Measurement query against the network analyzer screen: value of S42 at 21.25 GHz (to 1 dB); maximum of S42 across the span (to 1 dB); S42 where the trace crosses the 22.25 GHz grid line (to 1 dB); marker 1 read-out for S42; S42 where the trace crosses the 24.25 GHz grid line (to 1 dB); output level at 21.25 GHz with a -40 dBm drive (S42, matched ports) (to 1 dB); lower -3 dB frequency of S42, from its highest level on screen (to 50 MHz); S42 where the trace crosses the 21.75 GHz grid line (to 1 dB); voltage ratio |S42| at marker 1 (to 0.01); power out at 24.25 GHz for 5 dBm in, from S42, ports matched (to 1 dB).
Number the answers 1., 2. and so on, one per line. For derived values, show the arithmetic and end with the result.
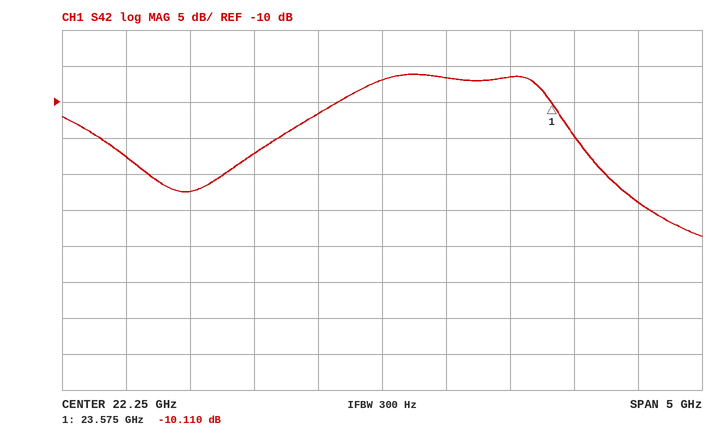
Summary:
1. -17 dB
2. -6 dB
3. -7 dB
4. -10.110 dB
5. -24 dB
6. -40 dBm + (-17 dB) = -57 dBm
7. 22.00 GHz
8. -12 dB
9. 10^(-10.11/20) ≈ 0.31
10. 5 dBm + (-24 dB) = -19 dBm
